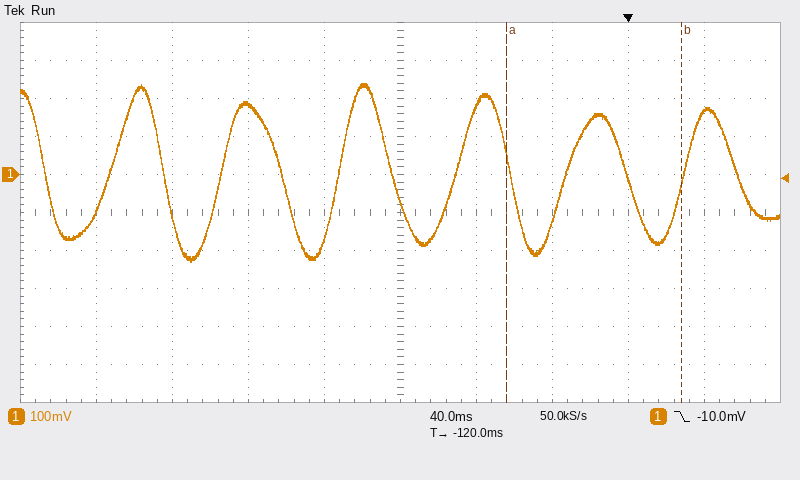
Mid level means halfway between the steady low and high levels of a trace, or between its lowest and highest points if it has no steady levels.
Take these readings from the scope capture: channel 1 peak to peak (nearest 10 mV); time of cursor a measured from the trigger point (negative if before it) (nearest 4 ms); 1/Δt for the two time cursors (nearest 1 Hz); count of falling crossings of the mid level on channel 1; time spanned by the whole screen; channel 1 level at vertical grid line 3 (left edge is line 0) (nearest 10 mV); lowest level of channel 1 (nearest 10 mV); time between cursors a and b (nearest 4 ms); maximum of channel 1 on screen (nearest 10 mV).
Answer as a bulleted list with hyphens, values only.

- 470 mV
- -64 ms
- 11 Hz
- 7
- 400 ms
- 180 mV
- -230 mV
- 92 ms
- 240 mV
